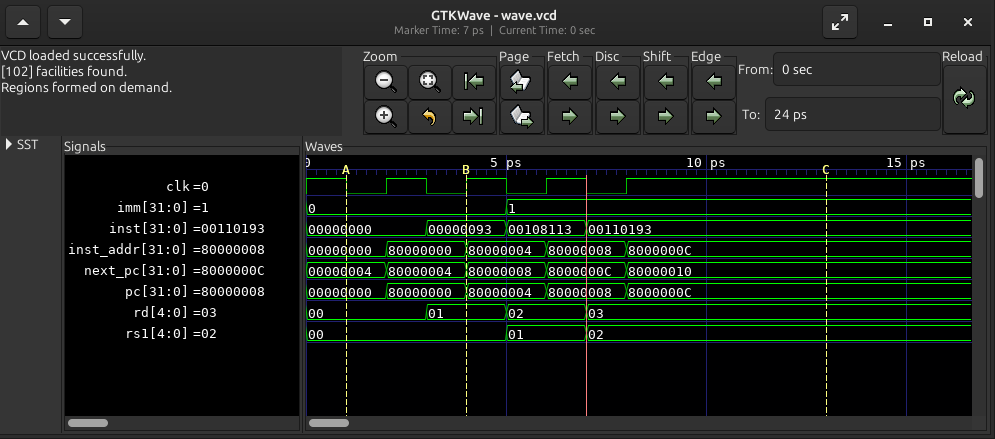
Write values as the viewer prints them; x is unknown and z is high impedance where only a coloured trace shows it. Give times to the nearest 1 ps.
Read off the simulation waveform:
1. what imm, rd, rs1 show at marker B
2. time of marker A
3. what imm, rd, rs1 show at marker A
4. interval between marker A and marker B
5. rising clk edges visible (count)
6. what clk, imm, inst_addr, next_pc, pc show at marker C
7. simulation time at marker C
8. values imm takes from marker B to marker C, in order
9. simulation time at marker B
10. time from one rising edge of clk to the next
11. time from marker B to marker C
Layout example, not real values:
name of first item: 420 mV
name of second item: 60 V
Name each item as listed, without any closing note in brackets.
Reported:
what imm, rd, rs1 show at marker B: imm=0, rd=01, rs1=00
time of marker A: 1 ps
what imm, rd, rs1 show at marker A: imm=0, rd=00, rs1=00
interval between marker A and marker B: 3 ps
rising clk edges visible: 4
what clk, imm, inst_addr, next_pc, pc show at marker C: clk=1, imm=1, inst_addr=8000000C, next_pc=80000010, pc=8000000C
simulation time at marker C: 13 ps
values imm takes from marker B to marker C, in order: 0, 1
simulation time at marker B: 4 ps
time from one rising edge of clk to the next: 2 ps
time from marker B to marker C: 9 ps
